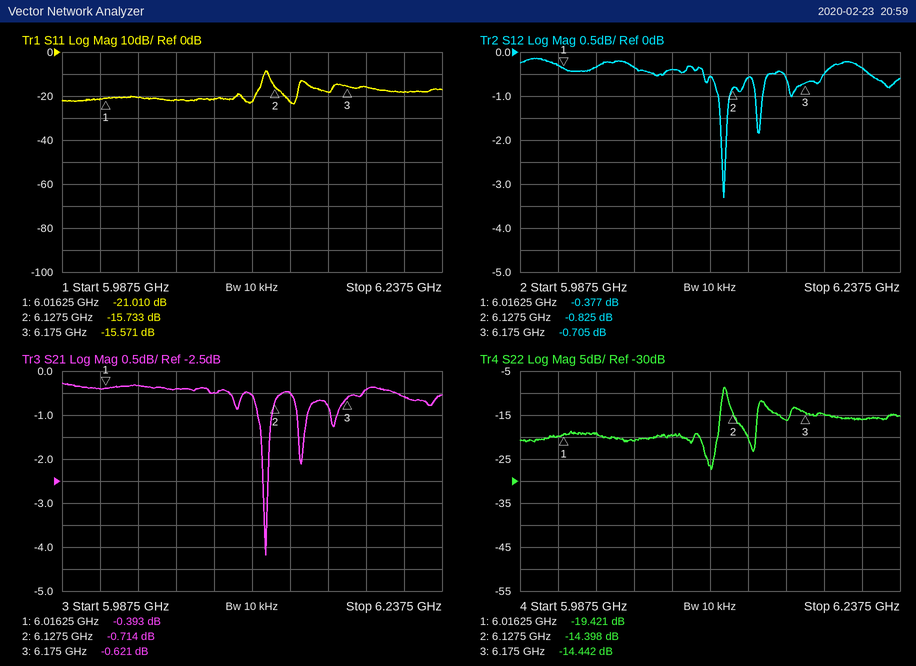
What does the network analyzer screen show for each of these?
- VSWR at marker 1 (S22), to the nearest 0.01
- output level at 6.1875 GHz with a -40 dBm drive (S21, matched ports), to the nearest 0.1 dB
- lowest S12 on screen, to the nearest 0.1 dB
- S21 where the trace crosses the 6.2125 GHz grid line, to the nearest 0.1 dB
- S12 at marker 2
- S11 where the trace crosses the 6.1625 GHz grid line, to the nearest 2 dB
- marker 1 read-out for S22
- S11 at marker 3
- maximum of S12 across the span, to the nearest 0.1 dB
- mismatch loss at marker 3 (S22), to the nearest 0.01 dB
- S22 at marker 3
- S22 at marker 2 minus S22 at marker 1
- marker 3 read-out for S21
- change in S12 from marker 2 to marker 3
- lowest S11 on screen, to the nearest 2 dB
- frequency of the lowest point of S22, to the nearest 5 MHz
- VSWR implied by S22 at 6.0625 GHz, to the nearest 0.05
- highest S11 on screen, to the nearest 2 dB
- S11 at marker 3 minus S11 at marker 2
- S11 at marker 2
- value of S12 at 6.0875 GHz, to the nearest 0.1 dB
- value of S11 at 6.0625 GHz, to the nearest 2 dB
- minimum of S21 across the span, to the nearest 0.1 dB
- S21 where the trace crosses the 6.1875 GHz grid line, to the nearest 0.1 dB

1.24
-40.4 dBm
-3.3 dB
-0.6 dB
-0.825 dB
-18 dB
-19.421 dB
-15.571 dB
-0.1 dB
0.16 dB
-14.442 dB
5.023 dB
-0.621 dB
0.120 dB
-24 dB
6.115 GHz
1.20
-8 dB
0.162 dB
-15.733 dB
-0.4 dB
-22 dB
-4.2 dB
-0.4 dB
